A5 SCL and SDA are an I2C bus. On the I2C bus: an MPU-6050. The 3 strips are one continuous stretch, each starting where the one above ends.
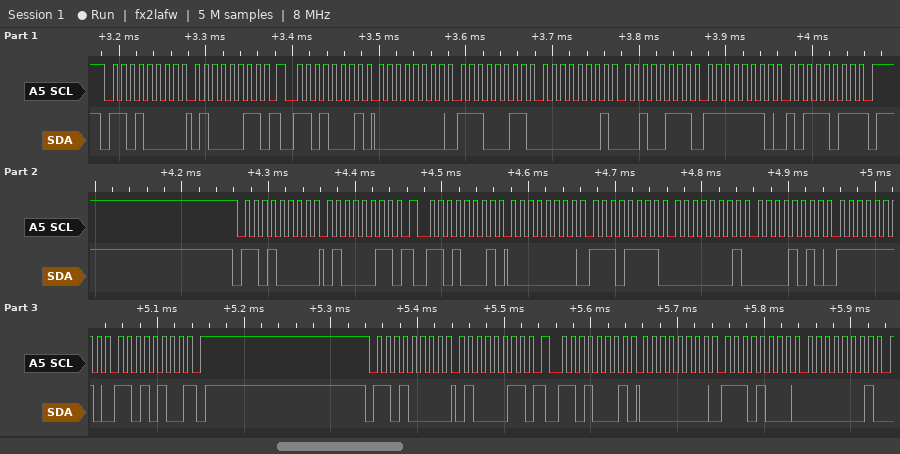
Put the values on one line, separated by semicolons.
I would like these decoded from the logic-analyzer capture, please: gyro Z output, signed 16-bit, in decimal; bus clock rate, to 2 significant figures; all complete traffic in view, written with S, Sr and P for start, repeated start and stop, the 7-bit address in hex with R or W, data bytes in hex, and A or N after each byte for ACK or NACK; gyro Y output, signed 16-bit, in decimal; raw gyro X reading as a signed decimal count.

-325; 100 kHz; S 68W A 43 A Sr 68R A 00 A E3 A 01 A 27 A FE A BB N P S 68W A 43 A Sr 68R A 00 A EF A 01 A 0A A FE A D4 N P S 68W A 43 A Sr 68R A 00 A E8 A 01 A; 295; 227
